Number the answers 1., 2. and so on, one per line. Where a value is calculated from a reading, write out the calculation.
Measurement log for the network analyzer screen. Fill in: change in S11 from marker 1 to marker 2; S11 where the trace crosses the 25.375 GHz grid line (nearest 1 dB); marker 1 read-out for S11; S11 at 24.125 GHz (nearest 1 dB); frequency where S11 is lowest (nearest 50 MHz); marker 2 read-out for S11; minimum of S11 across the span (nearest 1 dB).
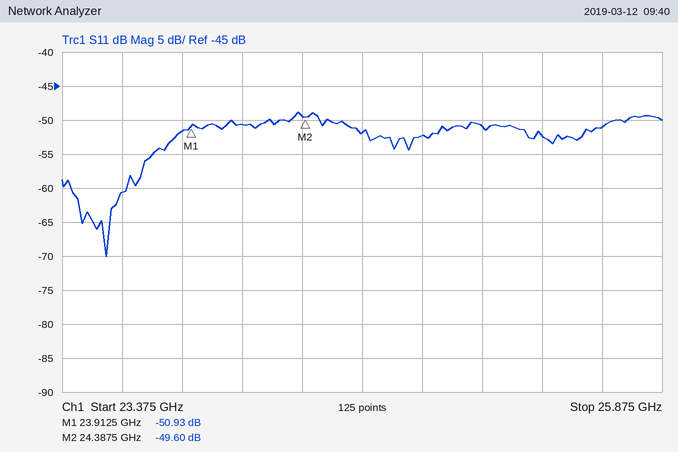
1. -49.6 − (-50.93) = 1.33 dB
2. -52 dB
3. -50.93 dB
4. -51 dB
5. 23.55 GHz
6. -49.60 dB
7. -70 dB
